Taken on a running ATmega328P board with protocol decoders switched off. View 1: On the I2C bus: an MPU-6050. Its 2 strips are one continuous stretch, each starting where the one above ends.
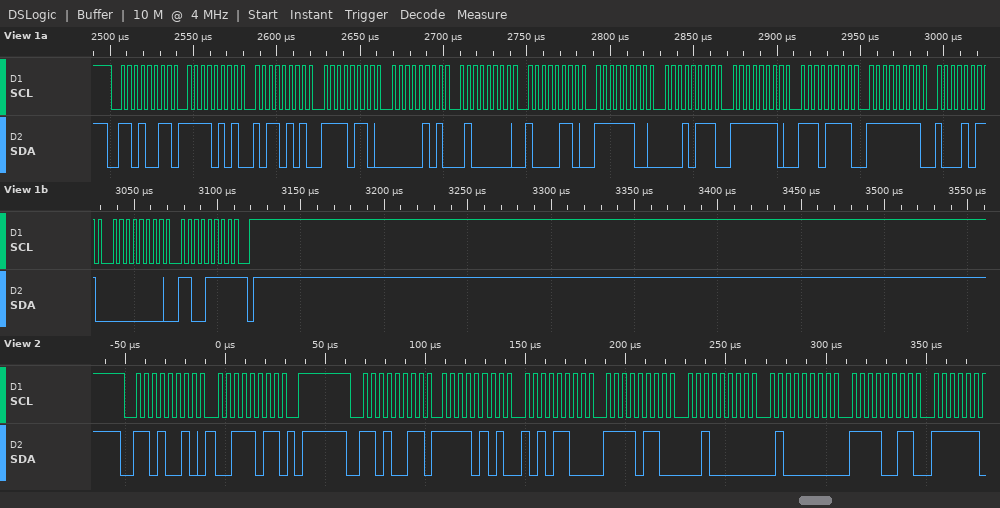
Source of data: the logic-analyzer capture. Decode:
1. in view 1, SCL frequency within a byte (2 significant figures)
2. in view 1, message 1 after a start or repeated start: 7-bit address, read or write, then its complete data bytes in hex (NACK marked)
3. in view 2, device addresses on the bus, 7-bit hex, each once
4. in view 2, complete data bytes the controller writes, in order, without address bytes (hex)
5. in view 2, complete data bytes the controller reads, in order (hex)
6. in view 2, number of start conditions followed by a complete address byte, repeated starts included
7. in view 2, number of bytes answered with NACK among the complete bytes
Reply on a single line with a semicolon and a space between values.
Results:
250 kHz; 0x69 read: F5 B5 F6 05 40 86 FC 17 FE EF FF 8B 00 CF NACK; 0x69; 3B; F5 AC F6 20 40 F3; 2; 0
